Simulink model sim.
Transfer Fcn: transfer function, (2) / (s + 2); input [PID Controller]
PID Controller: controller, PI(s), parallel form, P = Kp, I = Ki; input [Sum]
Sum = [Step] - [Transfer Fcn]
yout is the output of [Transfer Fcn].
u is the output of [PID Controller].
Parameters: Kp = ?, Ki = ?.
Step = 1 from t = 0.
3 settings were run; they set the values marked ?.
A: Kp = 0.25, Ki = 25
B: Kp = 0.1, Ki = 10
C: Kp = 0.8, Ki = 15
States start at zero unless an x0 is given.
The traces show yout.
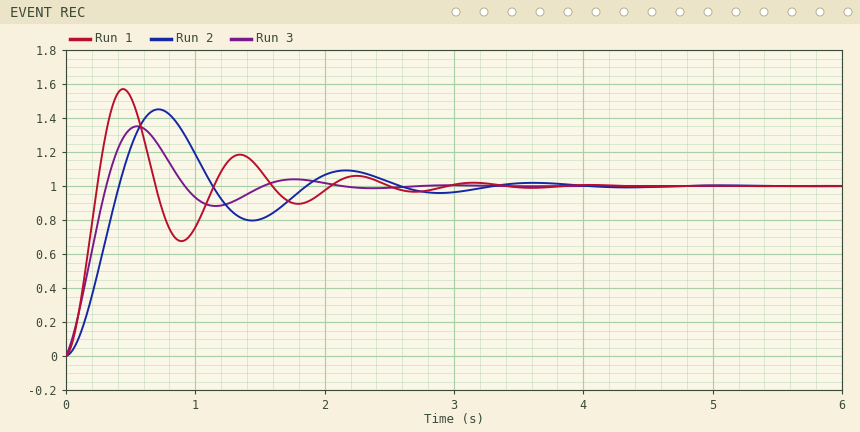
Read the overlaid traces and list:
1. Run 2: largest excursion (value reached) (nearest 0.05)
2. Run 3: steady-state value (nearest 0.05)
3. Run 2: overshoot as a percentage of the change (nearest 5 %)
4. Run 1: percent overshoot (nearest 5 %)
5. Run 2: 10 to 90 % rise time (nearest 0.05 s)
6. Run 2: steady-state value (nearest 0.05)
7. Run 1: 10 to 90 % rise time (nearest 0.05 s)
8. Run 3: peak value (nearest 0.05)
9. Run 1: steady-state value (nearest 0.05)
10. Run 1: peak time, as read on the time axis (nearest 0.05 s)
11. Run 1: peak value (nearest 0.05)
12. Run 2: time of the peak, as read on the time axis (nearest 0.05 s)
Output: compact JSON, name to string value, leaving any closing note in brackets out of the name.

{"Run 2: largest excursion (value reached)": "1.45", "Run 3: steady-state value": "1.00", "Run 2: overshoot as a percentage of the change": "45 %", "Run 1: percent overshoot": "55 %", "Run 2: 10 to 90 % rise time": "0.30 s", "Run 2: steady-state value": "1.00", "Run 1: 10 to 90 % rise time": "0.15 s", "Run 3: peak value": "1.35", "Run 1: steady-state value": "1.00", "Run 1: peak time, as read on the time axis": "0.45 s", "Run 1: peak value": "1.55", "Run 2: time of the peak, as read on the time axis": "0.70 s"}
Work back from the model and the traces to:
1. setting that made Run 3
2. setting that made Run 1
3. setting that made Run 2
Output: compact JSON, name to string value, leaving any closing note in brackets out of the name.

{"setting that made Run 3": "C", "setting that made Run 1": "A", "setting that made Run 2": "B"}
